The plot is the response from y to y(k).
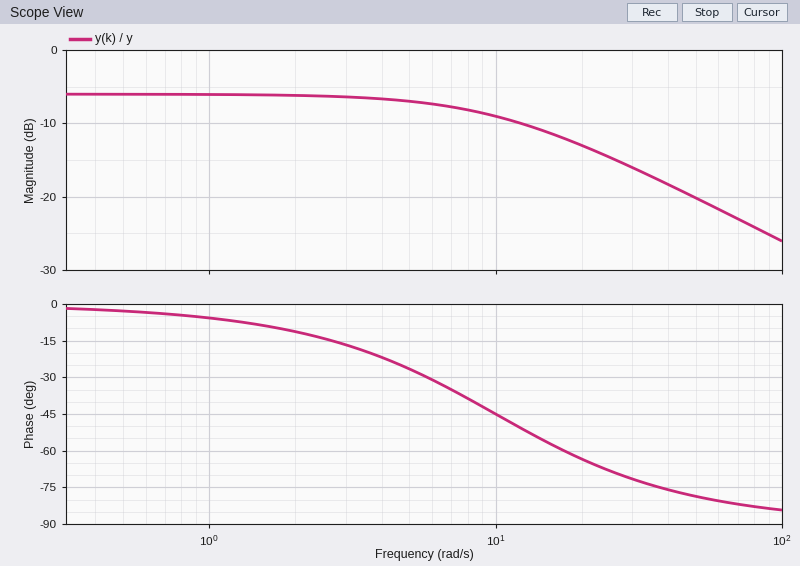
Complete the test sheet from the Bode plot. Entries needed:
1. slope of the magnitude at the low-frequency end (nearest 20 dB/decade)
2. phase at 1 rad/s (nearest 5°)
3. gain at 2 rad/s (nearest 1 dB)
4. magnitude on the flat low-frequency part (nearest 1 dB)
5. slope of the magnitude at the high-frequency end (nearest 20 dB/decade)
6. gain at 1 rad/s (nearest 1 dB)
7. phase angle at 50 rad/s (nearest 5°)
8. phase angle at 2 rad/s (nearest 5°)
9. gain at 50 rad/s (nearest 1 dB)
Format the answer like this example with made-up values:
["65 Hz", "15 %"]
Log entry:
["0 dB/decade", "-5°", "-6 dB", "-6 dB", "-20 dB/decade", "-6 dB", "-80°", "-10°", "-20 dB"]
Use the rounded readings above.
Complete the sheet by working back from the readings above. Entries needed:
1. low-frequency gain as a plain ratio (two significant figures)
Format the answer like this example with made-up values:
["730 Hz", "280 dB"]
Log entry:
["0.50"]
